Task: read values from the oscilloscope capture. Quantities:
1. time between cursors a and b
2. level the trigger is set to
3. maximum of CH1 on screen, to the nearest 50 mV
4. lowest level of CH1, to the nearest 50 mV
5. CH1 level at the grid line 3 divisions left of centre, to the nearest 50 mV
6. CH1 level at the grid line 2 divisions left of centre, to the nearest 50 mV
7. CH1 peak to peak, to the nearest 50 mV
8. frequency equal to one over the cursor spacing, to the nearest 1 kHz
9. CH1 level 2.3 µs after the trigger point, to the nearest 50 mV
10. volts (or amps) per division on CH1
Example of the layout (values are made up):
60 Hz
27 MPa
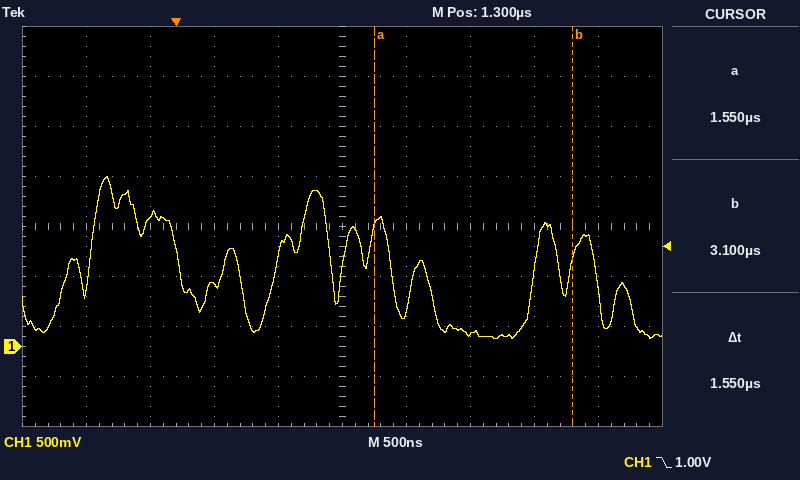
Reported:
1.55 µs
1.00 V
1.70 V
100 mV
1.30 V
600 mV
1.60 V
645 kHz
100 mV
500 mV
